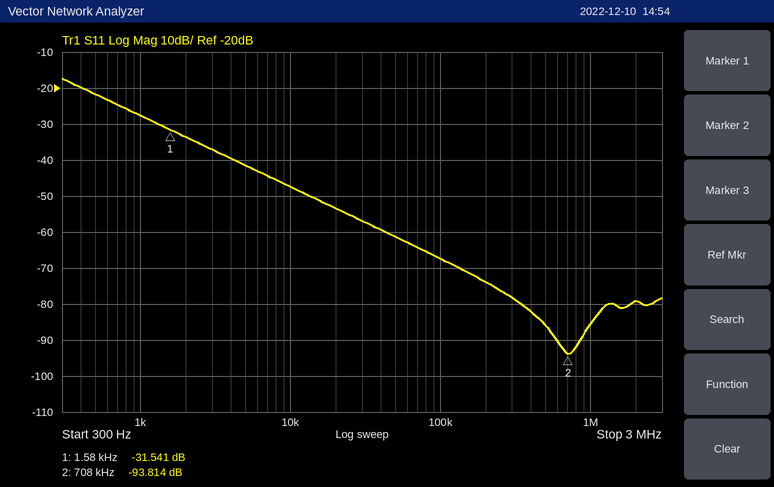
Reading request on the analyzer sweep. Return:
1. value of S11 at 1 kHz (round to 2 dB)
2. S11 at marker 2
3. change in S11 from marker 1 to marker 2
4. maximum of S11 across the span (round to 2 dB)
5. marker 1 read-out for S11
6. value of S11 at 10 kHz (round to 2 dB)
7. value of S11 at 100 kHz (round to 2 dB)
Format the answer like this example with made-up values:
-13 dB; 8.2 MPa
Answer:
-28 dB; -93.814 dB; -62.273 dB; -18 dB; -31.541 dB; -48 dB; -68 dB
